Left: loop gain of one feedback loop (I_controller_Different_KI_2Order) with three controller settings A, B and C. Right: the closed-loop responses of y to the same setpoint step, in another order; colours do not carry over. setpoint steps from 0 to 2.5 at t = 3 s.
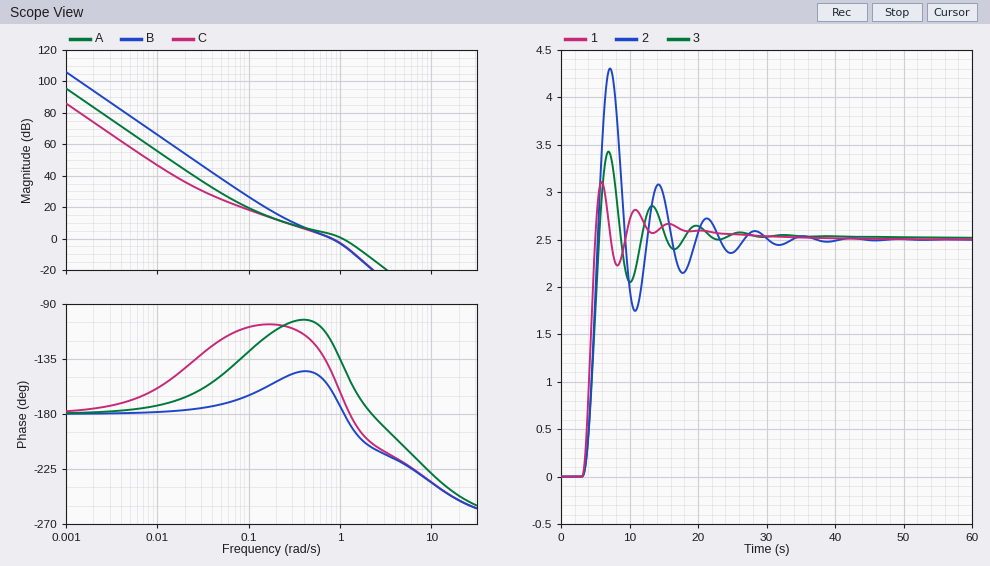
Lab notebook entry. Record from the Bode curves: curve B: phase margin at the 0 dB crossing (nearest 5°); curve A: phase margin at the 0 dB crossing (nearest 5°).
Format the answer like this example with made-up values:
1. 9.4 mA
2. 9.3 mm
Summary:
1. 20°
2. 40°
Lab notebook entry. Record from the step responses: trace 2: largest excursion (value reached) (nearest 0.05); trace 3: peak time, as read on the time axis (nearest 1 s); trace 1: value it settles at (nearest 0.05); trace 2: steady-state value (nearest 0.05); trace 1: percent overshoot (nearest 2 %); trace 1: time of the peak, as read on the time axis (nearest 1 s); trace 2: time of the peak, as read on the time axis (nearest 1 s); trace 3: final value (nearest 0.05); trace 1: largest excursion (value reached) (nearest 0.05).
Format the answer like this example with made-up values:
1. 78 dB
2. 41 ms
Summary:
1. 4.30
2. 7 s
3. 2.50
4. 2.50
5. 24 %
6. 6 s
7. 7 s
8. 2.50
9. 3.10
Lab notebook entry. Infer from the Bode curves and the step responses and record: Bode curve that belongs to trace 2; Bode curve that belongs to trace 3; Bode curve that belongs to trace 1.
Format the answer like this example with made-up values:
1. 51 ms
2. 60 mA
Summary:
1. B
2. C
3. A
